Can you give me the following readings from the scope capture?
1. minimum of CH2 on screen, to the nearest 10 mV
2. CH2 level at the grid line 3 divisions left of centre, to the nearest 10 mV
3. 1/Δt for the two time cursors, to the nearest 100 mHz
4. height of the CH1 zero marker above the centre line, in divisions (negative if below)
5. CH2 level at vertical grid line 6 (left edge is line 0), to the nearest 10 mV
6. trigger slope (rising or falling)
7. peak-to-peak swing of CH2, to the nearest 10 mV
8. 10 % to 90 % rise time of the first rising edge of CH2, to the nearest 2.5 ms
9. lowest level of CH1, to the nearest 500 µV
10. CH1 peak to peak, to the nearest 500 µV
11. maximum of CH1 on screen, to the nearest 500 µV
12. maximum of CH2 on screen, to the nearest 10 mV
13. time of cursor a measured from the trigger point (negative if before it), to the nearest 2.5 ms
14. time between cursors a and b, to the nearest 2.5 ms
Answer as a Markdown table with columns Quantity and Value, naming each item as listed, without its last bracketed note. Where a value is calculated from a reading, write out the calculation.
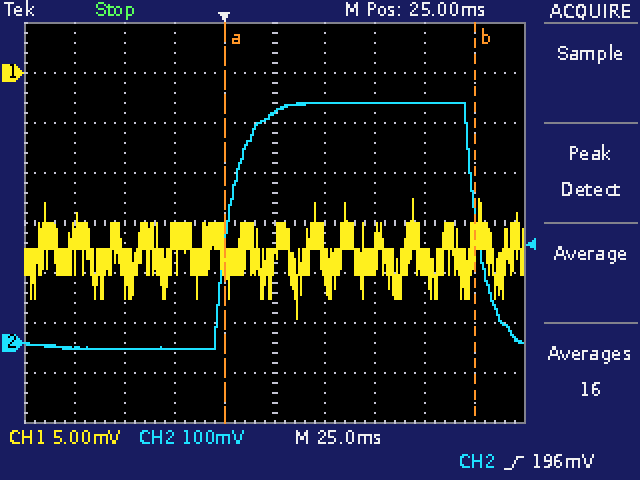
| Quantity | Value |
|---|---|
| minimum of CH2 on screen, to the nearest 10 mV | -10 mV |
| CH2 level at the grid line 3 divisions left of centre, to the nearest 10 mV | -10 mV |
| 1/Δt for the two time cursors, to the nearest 100 mHz | 1 / 125.0 ms ≈ 8.0 Hz |
| height of the CH1 zero marker above the centre line, in divisions | +3.0 div |
| CH2 level at vertical grid line 6 (left edge is line 0), to the nearest 10 mV | 480 mV |
| trigger slope | rising |
| peak-to-peak swing of CH2, to the nearest 10 mV | 480 mV − (-10 mV) = 490 mV |
| 10 % to 90 % rise time of the first rising edge of CH2, to the nearest 2.5 ms | 20.0 ms |
| lowest level of CH1, to the nearest 500 µV | -24.5 mV |
| CH1 peak to peak, to the nearest 500 µV | -12.5 mV − (-24.5 mV) = 12.0 mV |
| maximum of CH1 on screen, to the nearest 500 µV | -12.5 mV |
| maximum of CH2 on screen, to the nearest 10 mV | 480 mV |
| time of cursor a measured from the trigger point (negative if before it), to the nearest 2.5 ms | 0.0 ms |
| time between cursors a and b, to the nearest 2.5 ms | 125.0 ms |
